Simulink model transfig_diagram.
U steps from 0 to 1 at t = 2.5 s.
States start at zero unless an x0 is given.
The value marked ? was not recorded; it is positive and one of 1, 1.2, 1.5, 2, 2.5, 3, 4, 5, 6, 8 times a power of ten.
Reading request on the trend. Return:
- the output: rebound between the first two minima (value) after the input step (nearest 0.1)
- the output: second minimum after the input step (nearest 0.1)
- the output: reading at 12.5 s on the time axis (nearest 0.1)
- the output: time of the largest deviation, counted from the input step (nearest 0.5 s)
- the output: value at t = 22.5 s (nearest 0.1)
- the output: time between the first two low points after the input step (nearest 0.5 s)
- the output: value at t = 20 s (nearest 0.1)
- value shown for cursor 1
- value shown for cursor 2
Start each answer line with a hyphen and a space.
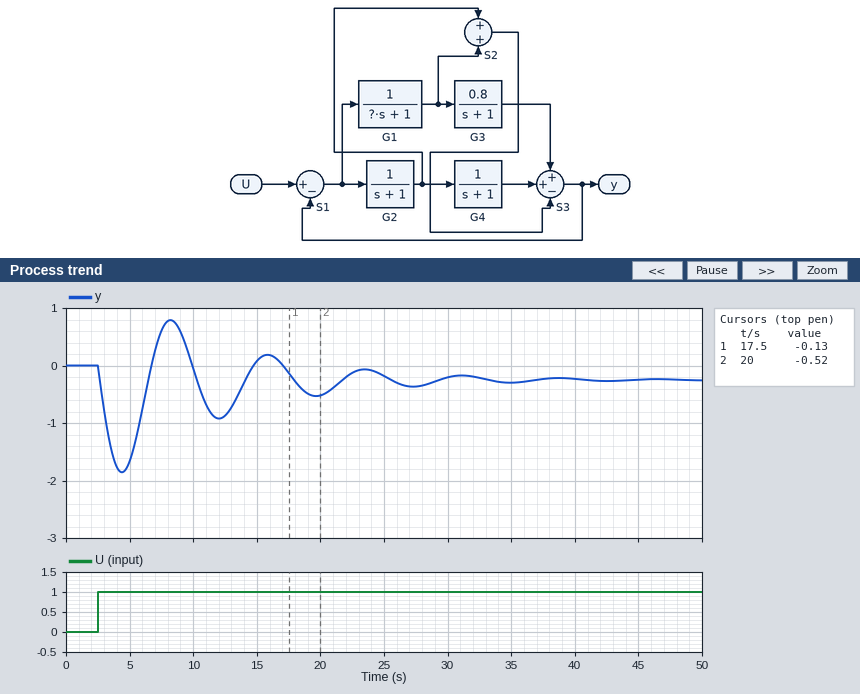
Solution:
- 0.8
- -0.9
- -0.9
- 2.0 s
- -0.1
- 7.5 s
- -0.5
- -0.13
- -0.52
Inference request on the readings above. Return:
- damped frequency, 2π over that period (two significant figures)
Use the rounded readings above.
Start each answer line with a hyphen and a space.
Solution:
- 0.84 rad/s
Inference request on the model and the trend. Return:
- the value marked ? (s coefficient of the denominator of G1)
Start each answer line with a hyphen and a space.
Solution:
- 1.5
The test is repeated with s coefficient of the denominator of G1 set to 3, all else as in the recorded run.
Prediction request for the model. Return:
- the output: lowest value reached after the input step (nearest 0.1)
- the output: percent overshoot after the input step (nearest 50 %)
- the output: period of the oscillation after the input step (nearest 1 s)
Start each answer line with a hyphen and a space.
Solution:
- -1.2
- 350 %
- 8 s
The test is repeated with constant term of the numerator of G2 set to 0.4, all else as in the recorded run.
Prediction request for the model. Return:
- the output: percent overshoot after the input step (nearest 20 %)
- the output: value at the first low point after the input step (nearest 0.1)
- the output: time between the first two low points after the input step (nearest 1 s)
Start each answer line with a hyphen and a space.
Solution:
- 260 %
- -0.9
- 9 s
